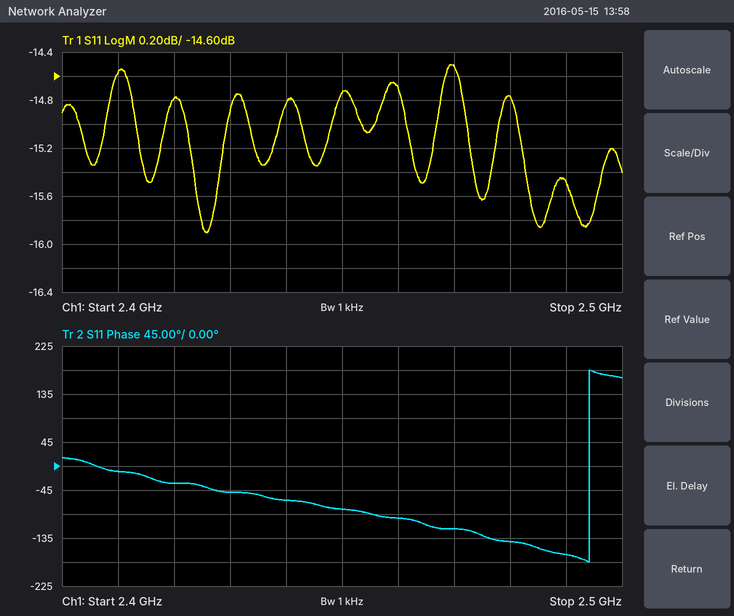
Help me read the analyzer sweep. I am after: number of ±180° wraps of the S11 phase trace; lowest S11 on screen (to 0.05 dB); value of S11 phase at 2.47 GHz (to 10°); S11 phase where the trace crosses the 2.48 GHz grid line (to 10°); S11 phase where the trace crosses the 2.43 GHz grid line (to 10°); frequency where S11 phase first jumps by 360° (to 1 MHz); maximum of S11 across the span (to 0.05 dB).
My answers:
1
-15.90 dB
-120°
-140°
-50°
2.494 GHz
-14.50 dB
